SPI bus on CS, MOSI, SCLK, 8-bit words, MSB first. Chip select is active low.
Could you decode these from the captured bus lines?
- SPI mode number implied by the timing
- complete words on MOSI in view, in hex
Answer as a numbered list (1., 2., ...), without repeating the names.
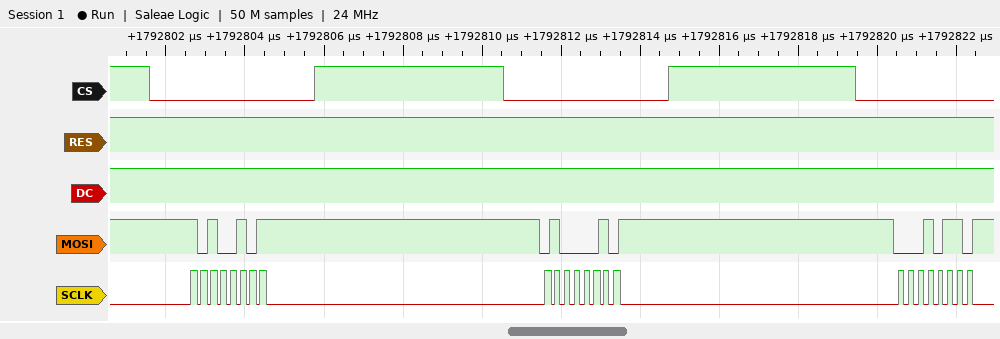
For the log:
1. 0
2. A5, 42, 16
